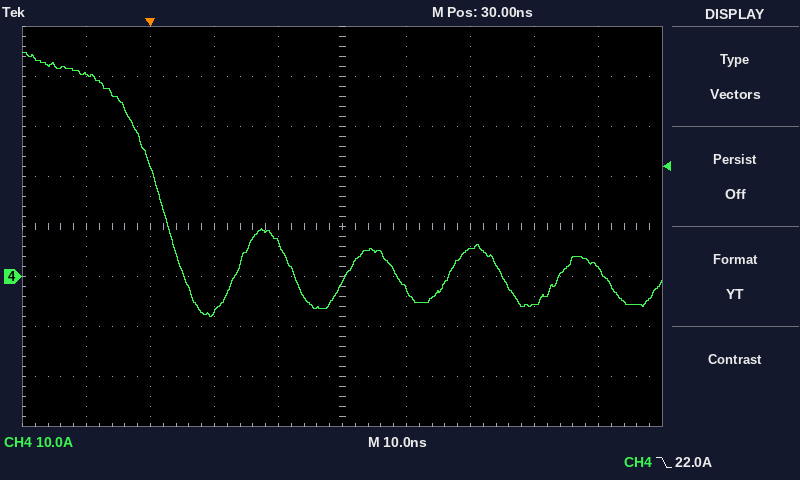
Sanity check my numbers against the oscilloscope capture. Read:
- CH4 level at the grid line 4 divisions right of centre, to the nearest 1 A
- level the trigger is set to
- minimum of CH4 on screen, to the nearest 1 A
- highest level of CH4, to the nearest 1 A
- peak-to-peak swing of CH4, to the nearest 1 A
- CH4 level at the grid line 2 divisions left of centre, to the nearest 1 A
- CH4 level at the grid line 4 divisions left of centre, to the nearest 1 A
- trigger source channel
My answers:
2 A
22.0 A
-8 A
45 A
53 A
-7 A
40 A
CH4
